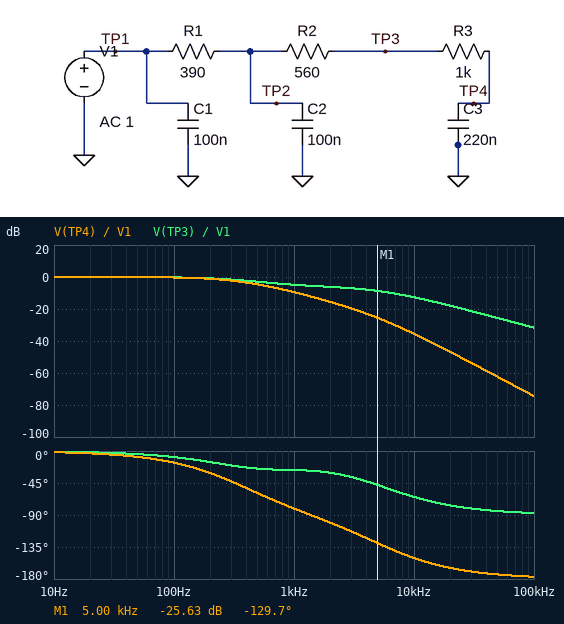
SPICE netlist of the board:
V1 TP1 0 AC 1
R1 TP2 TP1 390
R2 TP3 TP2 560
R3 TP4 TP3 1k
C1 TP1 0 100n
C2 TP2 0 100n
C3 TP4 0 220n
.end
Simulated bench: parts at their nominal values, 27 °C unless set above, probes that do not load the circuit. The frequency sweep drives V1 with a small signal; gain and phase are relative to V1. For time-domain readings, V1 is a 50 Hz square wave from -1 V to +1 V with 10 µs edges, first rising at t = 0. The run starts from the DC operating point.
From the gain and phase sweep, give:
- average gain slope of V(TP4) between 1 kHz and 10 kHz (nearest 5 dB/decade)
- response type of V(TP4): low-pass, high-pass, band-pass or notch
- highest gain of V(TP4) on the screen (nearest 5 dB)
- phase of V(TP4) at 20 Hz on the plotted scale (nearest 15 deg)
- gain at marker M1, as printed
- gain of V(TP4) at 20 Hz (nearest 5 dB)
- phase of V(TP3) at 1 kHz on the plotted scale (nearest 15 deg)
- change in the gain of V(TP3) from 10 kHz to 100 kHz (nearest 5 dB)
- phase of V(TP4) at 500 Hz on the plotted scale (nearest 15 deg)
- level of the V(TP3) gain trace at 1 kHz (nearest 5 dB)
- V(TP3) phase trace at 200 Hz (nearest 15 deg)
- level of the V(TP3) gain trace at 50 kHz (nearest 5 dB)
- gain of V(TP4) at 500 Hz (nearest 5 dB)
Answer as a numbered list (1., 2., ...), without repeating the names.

1. -25 dB/decade
2. low-pass
3. 0 dB
4. 0 deg
5. -25.63 dB
6. 0 dB
7. -30 deg
8. -20 dB
9. -60 deg
10. -5 dB
11. -15 deg
12. -25 dB
13. -5 dB
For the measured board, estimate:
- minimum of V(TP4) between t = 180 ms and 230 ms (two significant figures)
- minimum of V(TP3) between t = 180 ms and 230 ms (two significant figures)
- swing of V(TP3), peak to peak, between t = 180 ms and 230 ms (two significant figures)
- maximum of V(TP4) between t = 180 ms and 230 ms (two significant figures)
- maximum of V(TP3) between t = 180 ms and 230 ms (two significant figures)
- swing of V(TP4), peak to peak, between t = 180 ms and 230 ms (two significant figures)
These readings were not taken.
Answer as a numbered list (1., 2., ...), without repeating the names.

1. -1.0 V
2. -1.0 V
3. 2.0 V
4. 1.0 V
5. 1.0 V
6. 2.0 V
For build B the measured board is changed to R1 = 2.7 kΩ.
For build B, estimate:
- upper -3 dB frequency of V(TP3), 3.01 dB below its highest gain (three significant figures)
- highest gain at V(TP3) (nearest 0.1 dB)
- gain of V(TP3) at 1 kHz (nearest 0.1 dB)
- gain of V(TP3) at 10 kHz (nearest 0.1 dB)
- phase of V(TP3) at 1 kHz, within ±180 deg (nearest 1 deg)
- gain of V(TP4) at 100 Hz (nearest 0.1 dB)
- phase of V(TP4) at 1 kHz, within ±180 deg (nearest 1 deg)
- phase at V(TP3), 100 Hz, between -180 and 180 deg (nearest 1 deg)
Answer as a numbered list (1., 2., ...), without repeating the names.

1. 146 Hz
2. 0 dB
3. -13.5 dB
4. -28.6 dB
5. -55 deg
6. -1.8 dB
7. -109 deg
8. -30 deg
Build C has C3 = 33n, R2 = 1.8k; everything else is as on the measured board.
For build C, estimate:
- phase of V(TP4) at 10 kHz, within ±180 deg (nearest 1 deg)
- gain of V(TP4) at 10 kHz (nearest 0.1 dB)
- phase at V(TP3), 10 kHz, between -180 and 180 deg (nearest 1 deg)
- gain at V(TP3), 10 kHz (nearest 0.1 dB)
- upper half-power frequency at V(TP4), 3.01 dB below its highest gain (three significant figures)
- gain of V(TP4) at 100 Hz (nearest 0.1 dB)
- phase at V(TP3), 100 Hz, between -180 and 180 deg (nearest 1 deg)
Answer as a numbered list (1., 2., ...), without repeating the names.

1. -146 deg
2. -24.1 dB
3. -81 deg
4. -16.9 dB
5. 1.32 kHz
6. 0 dB
7. -4 deg
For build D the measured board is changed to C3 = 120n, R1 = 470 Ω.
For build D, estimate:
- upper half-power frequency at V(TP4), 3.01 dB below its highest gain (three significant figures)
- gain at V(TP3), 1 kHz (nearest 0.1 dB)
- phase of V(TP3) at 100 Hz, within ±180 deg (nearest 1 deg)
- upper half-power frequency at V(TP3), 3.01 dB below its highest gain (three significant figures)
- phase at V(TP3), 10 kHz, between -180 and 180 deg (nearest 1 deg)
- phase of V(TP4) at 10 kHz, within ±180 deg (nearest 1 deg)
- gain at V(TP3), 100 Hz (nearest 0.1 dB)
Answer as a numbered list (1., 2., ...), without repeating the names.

1. 610 Hz
2. -3.8 dB
3. -6 deg
4. 796 Hz
5. -69 deg
6. -152 deg
7. -0.1 dB
